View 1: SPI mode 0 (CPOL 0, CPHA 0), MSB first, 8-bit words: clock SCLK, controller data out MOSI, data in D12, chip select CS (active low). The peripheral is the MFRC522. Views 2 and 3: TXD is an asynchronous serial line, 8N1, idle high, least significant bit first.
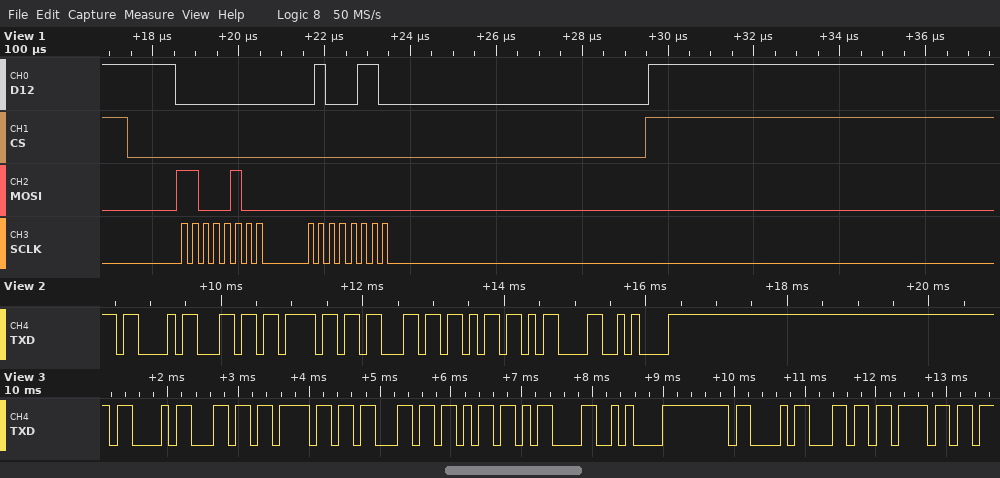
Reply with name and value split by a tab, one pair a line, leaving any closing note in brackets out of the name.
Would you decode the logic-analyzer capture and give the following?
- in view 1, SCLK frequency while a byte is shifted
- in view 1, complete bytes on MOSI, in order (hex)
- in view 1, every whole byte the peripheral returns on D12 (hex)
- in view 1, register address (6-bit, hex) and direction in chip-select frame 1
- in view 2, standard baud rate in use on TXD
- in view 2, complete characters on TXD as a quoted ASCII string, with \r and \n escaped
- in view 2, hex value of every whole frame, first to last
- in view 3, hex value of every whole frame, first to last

in view 1, SCLK frequency while a byte is shifted	4 MHz
in view 1, complete bytes on MOSI, in order	0xC4 0x00
in view 1, every whole byte the peripheral returns on D12	0x00 0x46
in view 1, register address (6-bit, hex) and direction in chip-select frame 1	0x22 read
in view 2, standard baud rate in use on TXD	9600 baud
in view 2, complete characters on TXD as a quoted ASCII string, with \r and \n escaped	"Clock\r\n"
in view 2, hex value of every whole frame, first to last	43 6C 6F 63 6B 0D 0A
in view 3, hex value of every whole frame, first to last	43 6C 6F 63 6B 0D 0A 43 6C 6F
